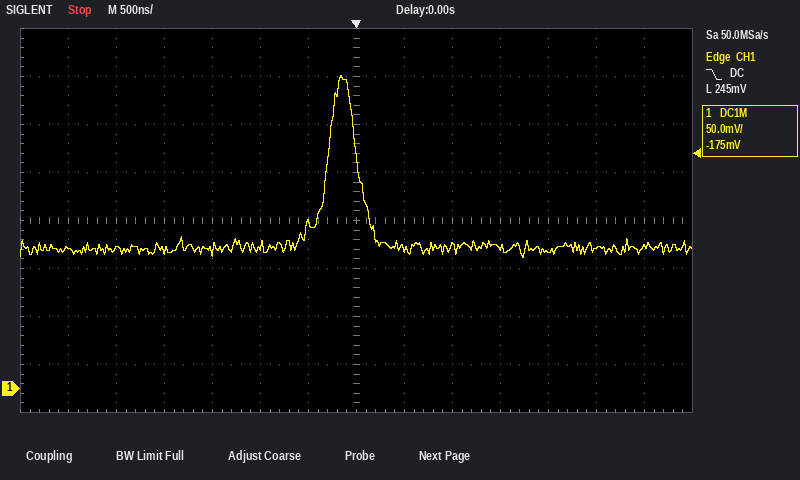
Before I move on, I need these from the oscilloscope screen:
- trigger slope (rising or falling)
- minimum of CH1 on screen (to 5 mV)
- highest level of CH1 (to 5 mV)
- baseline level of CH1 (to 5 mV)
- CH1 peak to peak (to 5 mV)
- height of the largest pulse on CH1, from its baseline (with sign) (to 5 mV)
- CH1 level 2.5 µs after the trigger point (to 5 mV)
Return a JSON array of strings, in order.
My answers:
["falling", "135 mV", "325 mV", "145 mV", "190 mV", "+180 mV", "145 mV"]
